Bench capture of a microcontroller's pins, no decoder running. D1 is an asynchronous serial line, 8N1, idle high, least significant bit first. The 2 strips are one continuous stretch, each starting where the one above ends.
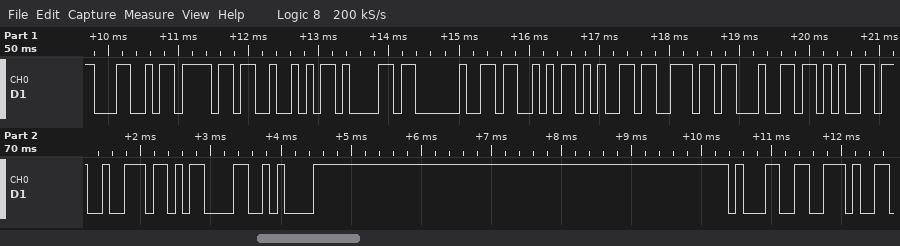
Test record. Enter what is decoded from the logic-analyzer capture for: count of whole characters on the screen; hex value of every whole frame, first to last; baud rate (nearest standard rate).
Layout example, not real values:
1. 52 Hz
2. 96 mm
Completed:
1. 15
2. 0x4C 0x6F 0x52 0x61 0x20 0x53 0x65 0x6E 0x64 0x65 0x72 0x0D 0x0A 0x31 0x2E
3. 9600 baud
